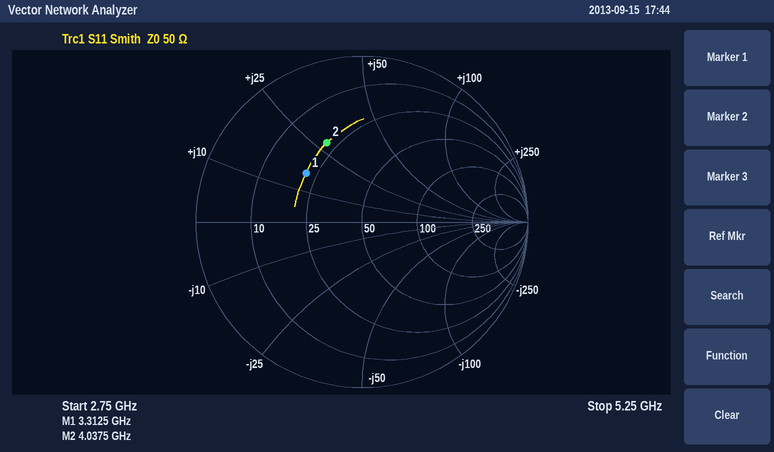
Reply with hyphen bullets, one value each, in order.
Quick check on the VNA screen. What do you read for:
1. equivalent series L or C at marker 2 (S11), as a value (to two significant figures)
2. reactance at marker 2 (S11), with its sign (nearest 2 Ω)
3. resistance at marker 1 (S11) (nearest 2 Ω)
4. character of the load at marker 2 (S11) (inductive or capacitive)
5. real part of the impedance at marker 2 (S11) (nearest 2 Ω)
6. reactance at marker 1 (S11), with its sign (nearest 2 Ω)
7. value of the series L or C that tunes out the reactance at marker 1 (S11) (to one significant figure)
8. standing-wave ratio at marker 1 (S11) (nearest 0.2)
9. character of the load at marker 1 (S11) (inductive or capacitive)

- 1.1 nH
- +28 Ω
- 22 Ω
- inductive
- 22 Ω
- +16 Ω
- 3 pF
- 2.6
- inductive
